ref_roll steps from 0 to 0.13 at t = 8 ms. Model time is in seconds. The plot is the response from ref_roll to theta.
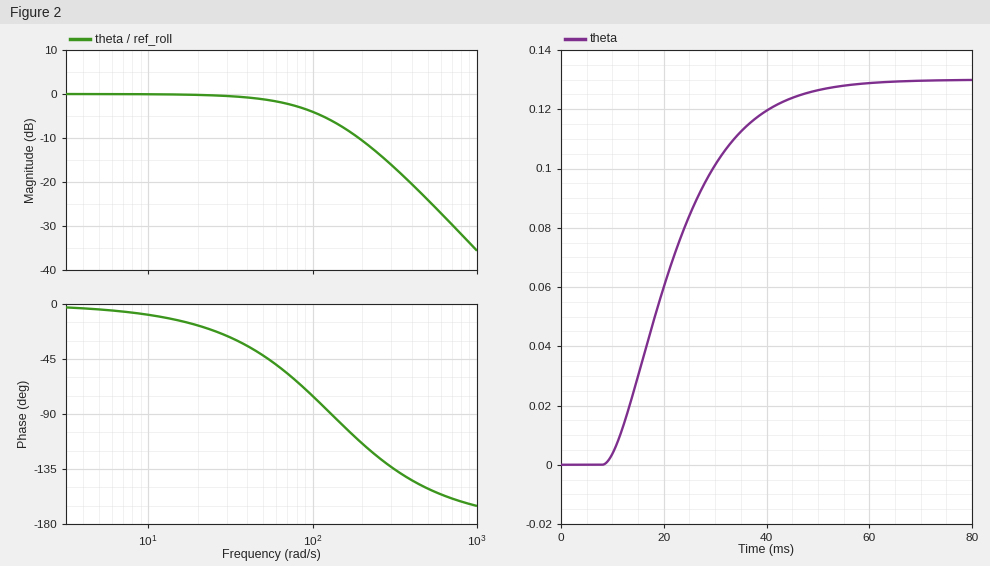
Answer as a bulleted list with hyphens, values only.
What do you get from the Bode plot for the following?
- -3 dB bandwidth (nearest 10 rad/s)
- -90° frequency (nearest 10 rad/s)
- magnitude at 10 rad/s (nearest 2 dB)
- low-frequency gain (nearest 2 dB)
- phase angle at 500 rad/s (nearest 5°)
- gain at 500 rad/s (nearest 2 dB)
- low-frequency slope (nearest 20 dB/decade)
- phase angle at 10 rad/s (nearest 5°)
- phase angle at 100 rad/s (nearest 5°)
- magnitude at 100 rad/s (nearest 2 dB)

- 80 rad/s
- 130 rad/s
- 0 dB
- 0 dB
- -150°
- -24 dB
- 0 dB/decade
- -10°
- -75°
- -4 dB
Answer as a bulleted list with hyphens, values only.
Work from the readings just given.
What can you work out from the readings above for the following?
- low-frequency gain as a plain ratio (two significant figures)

- 1.0
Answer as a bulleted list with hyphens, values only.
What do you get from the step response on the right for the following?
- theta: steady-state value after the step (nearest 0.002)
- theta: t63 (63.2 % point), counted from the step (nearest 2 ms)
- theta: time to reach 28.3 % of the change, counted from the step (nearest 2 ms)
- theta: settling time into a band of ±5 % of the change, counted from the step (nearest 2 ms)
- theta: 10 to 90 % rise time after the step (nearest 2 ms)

- 0.130
- 16 ms
- 8 ms
- 36 ms
- 26 ms
